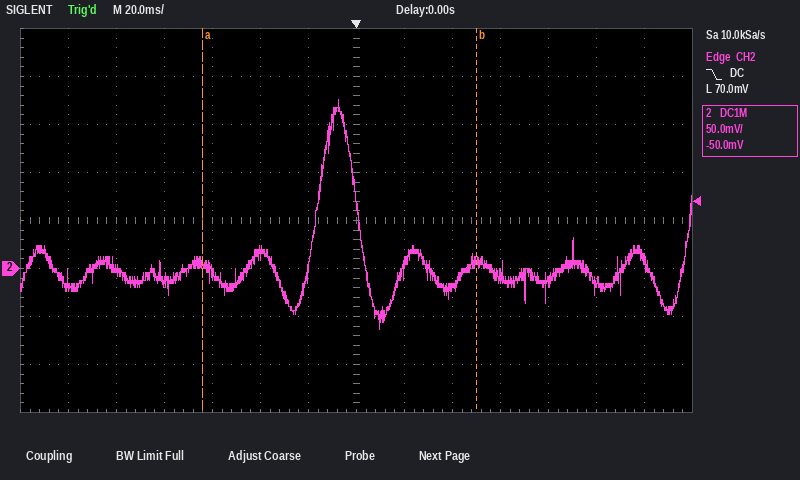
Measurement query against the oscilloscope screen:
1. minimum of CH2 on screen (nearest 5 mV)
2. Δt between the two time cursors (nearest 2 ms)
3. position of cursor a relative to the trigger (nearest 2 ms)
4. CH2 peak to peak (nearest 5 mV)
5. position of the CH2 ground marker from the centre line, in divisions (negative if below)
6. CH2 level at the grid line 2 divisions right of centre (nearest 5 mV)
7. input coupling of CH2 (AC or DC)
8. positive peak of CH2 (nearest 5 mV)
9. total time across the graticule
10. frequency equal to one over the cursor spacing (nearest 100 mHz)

-65 mV
114 ms
-64 ms
240 mV
-1.0 div
-20 mV
DC
175 mV
280 ms
8.8 Hz
